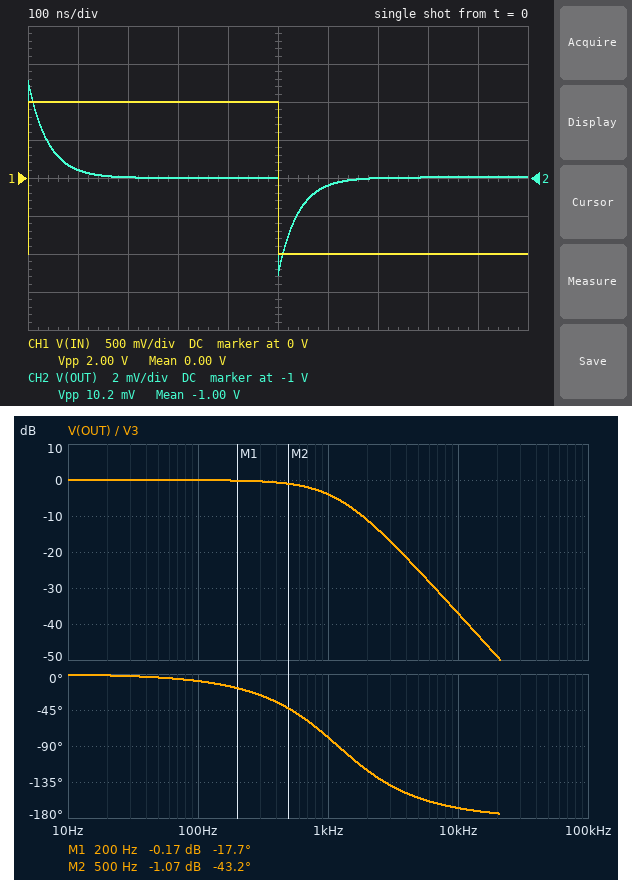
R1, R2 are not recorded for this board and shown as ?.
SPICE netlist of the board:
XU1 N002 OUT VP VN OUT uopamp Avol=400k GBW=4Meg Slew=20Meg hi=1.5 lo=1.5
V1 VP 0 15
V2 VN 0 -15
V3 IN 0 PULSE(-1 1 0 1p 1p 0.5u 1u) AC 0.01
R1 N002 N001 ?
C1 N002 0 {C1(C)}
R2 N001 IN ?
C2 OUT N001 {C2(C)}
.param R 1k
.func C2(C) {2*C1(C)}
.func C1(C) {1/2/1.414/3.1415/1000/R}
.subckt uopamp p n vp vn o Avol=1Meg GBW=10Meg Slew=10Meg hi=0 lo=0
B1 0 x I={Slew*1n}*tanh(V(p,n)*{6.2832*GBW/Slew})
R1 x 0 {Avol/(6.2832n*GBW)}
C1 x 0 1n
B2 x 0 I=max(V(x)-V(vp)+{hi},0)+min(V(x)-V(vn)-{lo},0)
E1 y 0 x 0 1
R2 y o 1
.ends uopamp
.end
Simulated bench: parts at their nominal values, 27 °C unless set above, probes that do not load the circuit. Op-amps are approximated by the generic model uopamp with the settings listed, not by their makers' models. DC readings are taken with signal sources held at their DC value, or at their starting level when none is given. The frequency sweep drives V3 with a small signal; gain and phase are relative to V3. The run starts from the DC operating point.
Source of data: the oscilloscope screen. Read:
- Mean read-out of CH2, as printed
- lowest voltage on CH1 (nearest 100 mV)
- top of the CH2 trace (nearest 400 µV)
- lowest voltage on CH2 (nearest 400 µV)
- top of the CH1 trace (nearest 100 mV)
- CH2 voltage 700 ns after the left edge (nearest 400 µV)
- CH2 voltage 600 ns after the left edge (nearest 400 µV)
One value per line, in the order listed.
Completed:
-1.00 V
-1.0 V
-994.8 mV
-1.0052 V
1.0 V
-1.0000 V
-1.0004 V
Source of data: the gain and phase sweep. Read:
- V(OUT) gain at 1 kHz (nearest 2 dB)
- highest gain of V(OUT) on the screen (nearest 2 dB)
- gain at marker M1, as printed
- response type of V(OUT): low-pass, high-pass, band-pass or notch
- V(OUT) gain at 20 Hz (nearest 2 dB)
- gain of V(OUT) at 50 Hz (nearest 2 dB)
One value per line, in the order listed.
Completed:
-4 dB
0 dB
-0.17 dB
low-pass
0 dB
0 dB
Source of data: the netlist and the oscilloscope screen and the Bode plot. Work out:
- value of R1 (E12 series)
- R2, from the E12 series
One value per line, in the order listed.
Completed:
1.8 kΩ
390 Ω
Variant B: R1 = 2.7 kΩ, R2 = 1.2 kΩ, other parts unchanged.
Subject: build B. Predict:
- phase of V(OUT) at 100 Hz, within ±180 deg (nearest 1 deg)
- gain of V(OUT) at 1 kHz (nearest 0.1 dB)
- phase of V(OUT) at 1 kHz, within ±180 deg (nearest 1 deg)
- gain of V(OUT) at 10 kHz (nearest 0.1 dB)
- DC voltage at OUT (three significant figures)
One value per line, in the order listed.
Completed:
-16 deg
-11.0 dB
-129 deg
-50.2 dB
-1.00 V
